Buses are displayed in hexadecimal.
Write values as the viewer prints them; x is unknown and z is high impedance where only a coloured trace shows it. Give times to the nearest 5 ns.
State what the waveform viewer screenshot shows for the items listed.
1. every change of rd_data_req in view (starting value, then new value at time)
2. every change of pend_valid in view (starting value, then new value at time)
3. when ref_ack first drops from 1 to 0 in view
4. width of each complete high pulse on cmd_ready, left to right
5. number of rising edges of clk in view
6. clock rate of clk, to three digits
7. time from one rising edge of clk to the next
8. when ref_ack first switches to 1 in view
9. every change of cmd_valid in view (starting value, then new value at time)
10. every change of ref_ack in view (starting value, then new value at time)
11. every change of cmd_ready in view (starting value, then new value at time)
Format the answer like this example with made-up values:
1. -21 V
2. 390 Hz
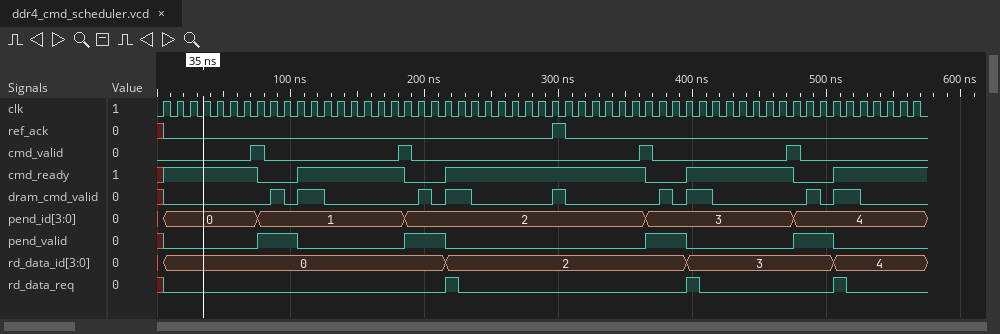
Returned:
1. x, 0 at 5 ns, 1 at 215 ns, 0 at 225 ns, 1 at 395 ns, 0 at 405 ns, 1 at 505 ns, 0 at 515 ns
2. x, 0 at 5 ns, 1 at 75 ns, 0 at 105 ns, 1 at 185 ns, 0 at 215 ns, 1 at 365 ns, 0 at 395 ns, 1 at 475 ns, 0 at 505 ns
3. 305 ns
4. 80 ns, 150 ns, 80 ns
5. 57
6. 100 MHz
7. 10 ns
8. 295 ns
9. 0, 1 at 70 ns, 0 at 80 ns, 1 at 180 ns, 0 at 190 ns, 1 at 360 ns, 0 at 370 ns, 1 at 470 ns, 0 at 480 ns
10. x, 0 at 5 ns, 1 at 295 ns, 0 at 305 ns
11. x, 1 at 5 ns, 0 at 75 ns, 1 at 105 ns, 0 at 185 ns, 1 at 215 ns, 0 at 365 ns, 1 at 395 ns, 0 at 475 ns, 1 at 505 ns
